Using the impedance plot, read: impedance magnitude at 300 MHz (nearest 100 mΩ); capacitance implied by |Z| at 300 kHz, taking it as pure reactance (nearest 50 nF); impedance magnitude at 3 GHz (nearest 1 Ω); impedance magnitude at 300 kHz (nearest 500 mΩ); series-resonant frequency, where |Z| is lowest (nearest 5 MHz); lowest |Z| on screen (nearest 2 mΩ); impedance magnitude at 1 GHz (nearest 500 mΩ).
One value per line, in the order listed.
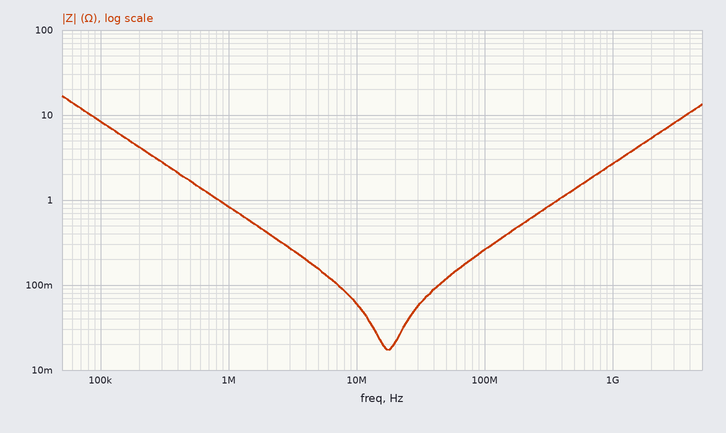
800 mΩ
200 nF
8 Ω
3.0 Ω
20 MHz
18 mΩ
2.5 Ω
